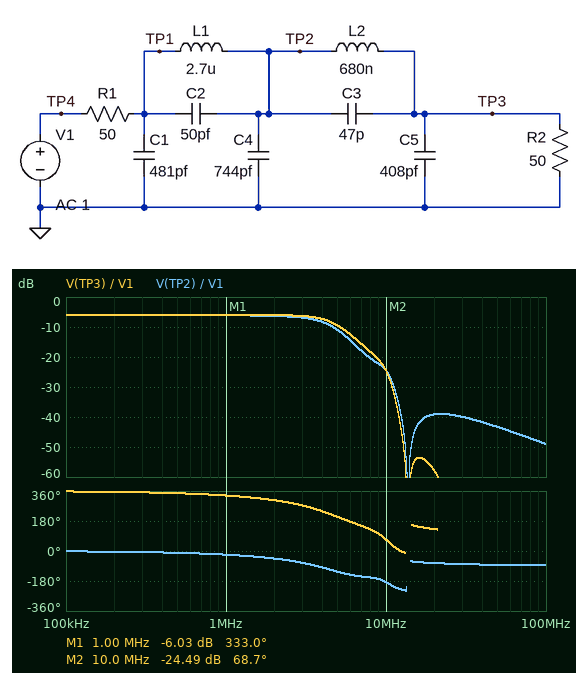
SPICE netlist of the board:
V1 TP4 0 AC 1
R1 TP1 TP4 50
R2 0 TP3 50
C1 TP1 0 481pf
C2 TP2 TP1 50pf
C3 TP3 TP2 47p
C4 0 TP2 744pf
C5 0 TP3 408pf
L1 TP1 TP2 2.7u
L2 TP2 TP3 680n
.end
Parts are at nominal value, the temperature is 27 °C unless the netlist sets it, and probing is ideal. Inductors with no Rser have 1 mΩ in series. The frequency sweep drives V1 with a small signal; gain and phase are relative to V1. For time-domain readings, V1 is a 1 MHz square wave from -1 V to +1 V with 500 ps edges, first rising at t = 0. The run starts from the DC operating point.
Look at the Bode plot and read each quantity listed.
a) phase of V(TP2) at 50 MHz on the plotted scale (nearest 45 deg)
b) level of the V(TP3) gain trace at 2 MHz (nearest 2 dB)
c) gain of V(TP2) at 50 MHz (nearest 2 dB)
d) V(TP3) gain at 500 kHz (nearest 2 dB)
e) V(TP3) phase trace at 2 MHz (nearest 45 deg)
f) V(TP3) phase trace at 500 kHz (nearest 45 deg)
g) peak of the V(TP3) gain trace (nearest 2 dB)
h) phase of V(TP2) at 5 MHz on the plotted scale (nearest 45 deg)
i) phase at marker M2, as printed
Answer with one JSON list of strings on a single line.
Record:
["-90 deg", "-6 dB", "-44 dB", "-6 dB", "315 deg", "360 deg", "-6 dB", "-135 deg", "68.7 deg"]
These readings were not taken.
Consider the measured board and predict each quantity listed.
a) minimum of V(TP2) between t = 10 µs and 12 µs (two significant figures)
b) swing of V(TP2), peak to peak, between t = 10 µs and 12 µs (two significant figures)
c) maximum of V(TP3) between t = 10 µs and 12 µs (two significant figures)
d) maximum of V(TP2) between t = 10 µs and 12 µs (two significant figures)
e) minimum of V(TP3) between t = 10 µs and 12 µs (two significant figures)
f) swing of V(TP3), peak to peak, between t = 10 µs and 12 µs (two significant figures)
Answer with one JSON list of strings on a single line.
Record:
["-560 mV", "1.1 V", "570 mV", "560 mV", "-570 mV", "1.1 V"]
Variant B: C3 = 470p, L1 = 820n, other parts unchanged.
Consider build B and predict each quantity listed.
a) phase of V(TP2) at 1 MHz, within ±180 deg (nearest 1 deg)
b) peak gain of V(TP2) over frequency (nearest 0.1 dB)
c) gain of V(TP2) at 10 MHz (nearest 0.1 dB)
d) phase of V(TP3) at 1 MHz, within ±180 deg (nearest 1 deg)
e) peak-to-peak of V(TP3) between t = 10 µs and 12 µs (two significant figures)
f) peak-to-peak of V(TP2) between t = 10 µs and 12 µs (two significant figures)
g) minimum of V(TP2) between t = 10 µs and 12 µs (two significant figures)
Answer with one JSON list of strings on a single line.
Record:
["-15 deg", "-1.1 dB", "-7.3 dB", "-20 deg", "1.2 V", "1.3 V", "-630 mV"]
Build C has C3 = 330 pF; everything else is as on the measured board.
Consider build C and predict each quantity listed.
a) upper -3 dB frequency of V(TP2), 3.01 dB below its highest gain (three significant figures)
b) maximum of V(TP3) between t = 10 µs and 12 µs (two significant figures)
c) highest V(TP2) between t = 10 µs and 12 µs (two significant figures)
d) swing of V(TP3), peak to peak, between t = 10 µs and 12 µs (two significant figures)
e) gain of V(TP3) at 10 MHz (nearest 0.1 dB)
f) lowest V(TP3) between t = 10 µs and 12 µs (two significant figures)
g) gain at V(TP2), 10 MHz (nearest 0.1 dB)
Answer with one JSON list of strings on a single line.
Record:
["4.36 MHz", "610 mV", "540 mV", "1.2 V", "-49.2 dB", "-610 mV", "-28.1 dB"]
